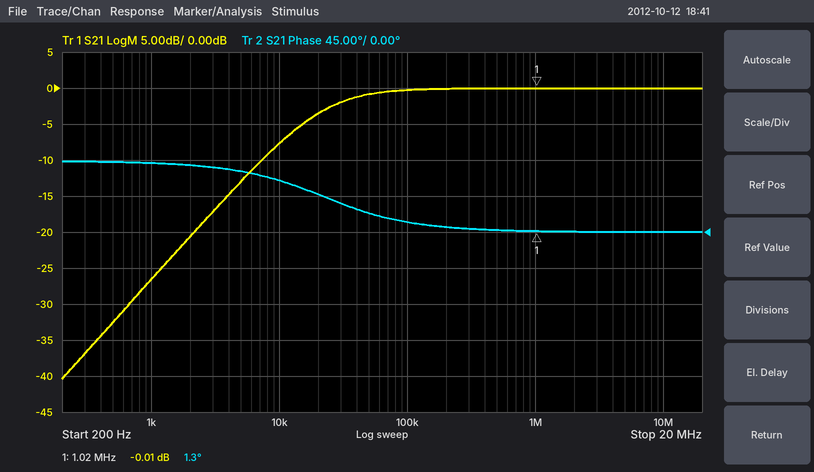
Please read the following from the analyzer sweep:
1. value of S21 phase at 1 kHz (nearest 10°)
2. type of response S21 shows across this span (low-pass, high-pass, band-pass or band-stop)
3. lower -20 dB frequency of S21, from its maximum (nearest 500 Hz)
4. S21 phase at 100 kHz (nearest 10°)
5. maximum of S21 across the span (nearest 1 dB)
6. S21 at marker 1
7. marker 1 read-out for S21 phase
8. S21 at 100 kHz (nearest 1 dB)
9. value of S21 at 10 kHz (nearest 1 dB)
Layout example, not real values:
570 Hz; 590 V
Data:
90°; high-pass; 2.0 kHz; 10°; 0 dB; -0.01 dB; 1.3°; 0 dB; -8 dB
